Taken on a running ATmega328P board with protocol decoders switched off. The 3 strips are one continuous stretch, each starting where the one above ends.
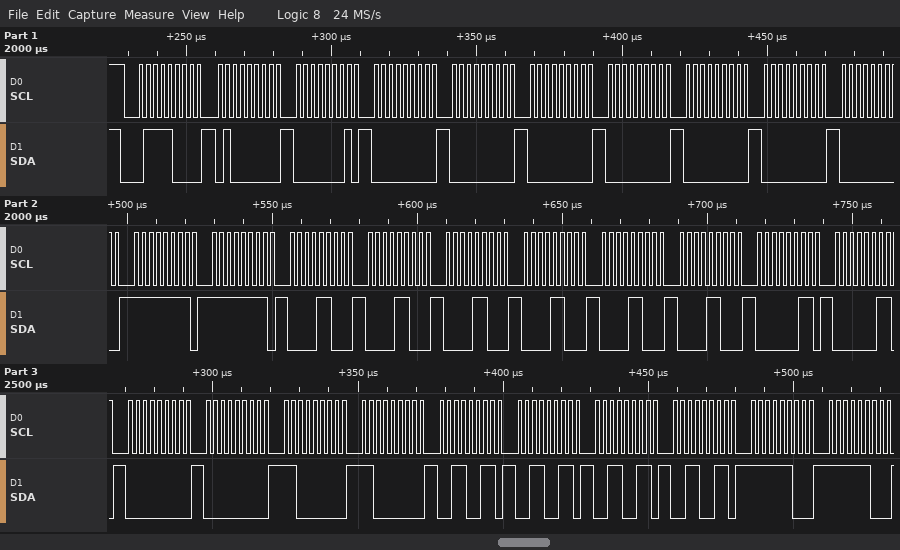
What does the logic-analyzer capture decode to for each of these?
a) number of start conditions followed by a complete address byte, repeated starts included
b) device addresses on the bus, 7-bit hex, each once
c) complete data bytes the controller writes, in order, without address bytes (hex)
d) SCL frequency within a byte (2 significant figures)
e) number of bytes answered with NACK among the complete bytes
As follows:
1
0x3C
40 01 00 00 00 00 00 00 00 FF FF 0C 0C 0C 0C 0C 0C 03 03 00 00 C0 C0 33 33 33 33 FC FC
400 kHz
0
